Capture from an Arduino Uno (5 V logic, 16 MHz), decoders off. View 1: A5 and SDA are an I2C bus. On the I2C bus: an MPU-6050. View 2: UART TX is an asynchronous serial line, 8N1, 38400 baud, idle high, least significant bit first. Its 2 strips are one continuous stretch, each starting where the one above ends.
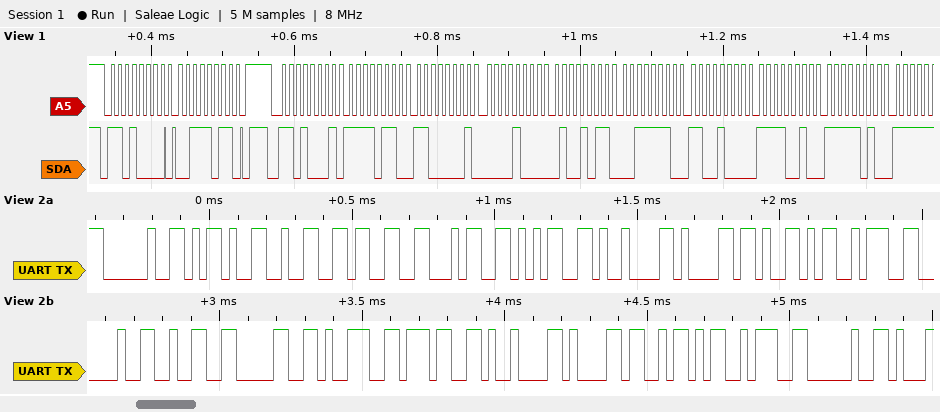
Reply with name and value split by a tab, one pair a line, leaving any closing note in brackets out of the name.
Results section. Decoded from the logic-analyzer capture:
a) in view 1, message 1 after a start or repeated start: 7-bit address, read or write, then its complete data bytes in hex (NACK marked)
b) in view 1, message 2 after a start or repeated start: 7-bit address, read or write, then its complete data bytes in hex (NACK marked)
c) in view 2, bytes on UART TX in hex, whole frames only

in view 1, message 1 after a start or repeated start: 7-bit address, read or write, then its complete data bytes in hex	0x68 write: 3B
in view 1, message 2 after a start or repeated start: 7-bit address, read or write, then its complete data bytes in hex	0x68 read: F6 C1 08 4B 3E C8 F2 FA
in view 2, bytes on UART TX in hex, whole frames only	20 2D 32 33 34 35 09 61 59 3A 20 32 30 39 37 09 61 5A 3A 20
